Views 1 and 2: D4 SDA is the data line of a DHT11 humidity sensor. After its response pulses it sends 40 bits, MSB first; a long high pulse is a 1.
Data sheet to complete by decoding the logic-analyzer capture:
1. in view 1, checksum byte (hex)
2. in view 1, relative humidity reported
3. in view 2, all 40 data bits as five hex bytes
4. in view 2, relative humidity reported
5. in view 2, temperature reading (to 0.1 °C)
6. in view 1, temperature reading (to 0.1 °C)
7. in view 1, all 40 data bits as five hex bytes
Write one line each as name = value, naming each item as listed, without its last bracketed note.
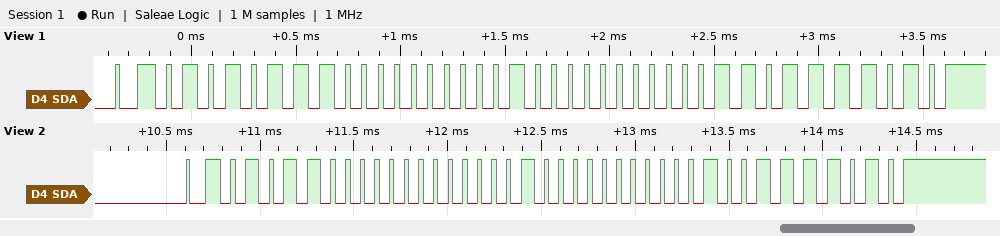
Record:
in view 1, checksum byte = 0x7A
in view 1, relative humidity reported = 87 %
in view 2, all 40 data bits as five hex bytes = 58 00 20 02 7A
in view 2, relative humidity reported = 88 %
in view 2, temperature reading = 32.2 °C
in view 1, temperature reading = 32.3 °C
in view 1, all 40 data bits as five hex bytes = 57 00 20 03 7A
